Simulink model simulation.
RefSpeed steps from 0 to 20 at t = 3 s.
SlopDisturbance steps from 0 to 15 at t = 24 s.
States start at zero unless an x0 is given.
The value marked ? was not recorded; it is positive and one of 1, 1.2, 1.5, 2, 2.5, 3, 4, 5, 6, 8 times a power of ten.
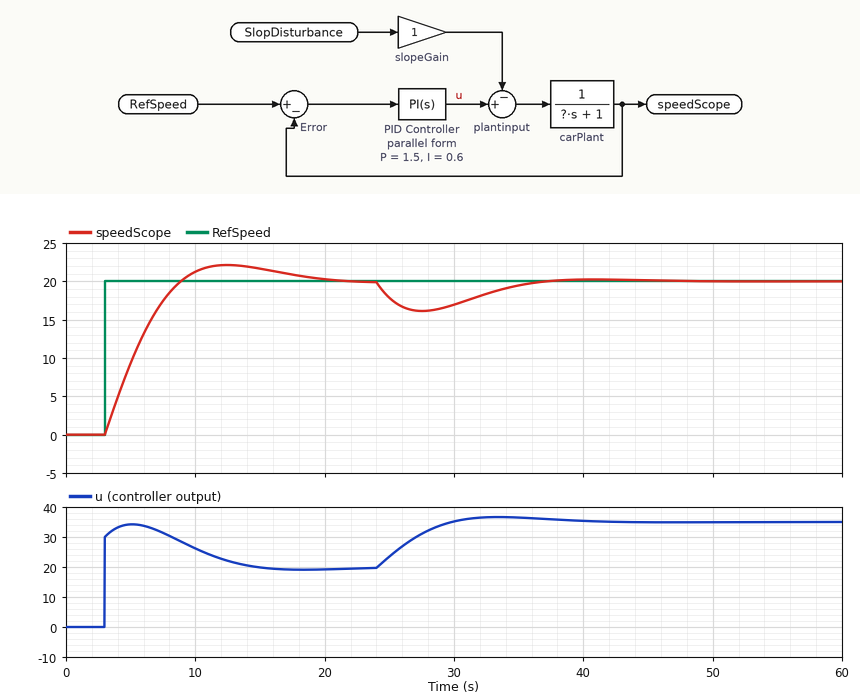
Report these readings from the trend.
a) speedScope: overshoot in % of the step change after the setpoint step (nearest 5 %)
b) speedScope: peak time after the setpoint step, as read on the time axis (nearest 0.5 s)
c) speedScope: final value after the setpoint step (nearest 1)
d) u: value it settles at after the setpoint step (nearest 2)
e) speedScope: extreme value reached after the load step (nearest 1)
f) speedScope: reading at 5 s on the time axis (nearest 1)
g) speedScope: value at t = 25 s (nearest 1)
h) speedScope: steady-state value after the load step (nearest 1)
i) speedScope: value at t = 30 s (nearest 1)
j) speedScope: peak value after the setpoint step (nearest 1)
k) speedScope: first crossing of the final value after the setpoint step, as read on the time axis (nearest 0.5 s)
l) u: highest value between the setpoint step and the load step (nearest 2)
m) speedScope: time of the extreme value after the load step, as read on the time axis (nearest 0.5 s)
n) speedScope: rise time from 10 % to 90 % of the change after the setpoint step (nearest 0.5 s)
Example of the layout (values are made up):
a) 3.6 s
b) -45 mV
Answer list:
a) 10 %
b) 12.5 s
c) 20
d) 20
e) 16
f) 9
g) 18
h) 20
i) 17
j) 22
k) 9.0 s
l) 34
m) 27.5 s
n) 4.5 s
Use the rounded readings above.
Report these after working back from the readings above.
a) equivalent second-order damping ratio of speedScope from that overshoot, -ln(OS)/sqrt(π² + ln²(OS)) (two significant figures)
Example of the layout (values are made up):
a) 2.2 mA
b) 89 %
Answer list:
a) 0.59
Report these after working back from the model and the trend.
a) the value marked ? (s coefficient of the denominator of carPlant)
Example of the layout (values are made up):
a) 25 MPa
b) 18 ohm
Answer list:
a) 6
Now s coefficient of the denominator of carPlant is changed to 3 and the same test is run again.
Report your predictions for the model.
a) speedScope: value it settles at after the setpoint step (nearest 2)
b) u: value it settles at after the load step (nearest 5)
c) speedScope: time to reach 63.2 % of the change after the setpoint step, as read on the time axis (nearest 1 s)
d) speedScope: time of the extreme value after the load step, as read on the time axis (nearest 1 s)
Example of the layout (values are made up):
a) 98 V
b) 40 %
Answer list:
a) 20
b) 35
c) 5 s
d) 26 s
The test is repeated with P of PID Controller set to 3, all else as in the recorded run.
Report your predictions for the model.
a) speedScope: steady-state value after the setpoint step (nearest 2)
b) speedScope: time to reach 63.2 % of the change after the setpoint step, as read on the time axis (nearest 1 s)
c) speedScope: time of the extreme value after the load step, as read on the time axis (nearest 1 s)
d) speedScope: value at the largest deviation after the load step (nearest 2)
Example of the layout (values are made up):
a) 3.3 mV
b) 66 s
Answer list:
a) 20
b) 5 s
c) 27 s
d) 18
